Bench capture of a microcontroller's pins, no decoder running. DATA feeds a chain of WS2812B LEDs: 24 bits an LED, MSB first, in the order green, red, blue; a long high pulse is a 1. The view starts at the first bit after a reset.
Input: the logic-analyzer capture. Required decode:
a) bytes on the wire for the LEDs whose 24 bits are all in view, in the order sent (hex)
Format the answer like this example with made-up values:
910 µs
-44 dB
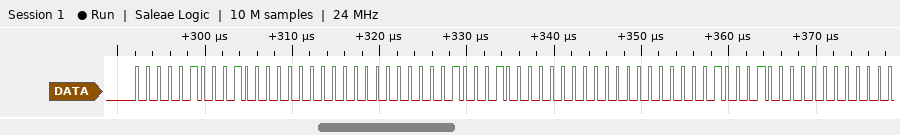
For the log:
04 40 00 04 40 00
